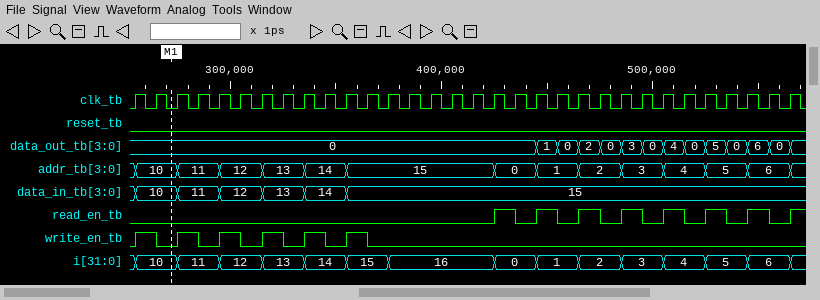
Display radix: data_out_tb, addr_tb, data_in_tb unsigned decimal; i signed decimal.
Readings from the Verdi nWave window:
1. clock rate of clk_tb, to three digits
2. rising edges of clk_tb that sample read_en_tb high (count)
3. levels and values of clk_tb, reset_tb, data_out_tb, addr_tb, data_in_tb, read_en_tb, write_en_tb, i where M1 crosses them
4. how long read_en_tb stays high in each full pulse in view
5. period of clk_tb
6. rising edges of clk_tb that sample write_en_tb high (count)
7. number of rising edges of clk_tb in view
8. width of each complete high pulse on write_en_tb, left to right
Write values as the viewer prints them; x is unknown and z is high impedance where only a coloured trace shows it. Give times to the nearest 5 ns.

100 MHz
7
clk_tb=0, reset_tb=0, data_out_tb=0, addr_tb=10, data_in_tb=10, read_en_tb=0, write_en_tb=0, i=10
10 ns, 10 ns, 10 ns, 10 ns, 10 ns, 10 ns, 10 ns
10 ns
6
32
10 ns, 10 ns, 10 ns, 10 ns, 10 ns, 10 ns
